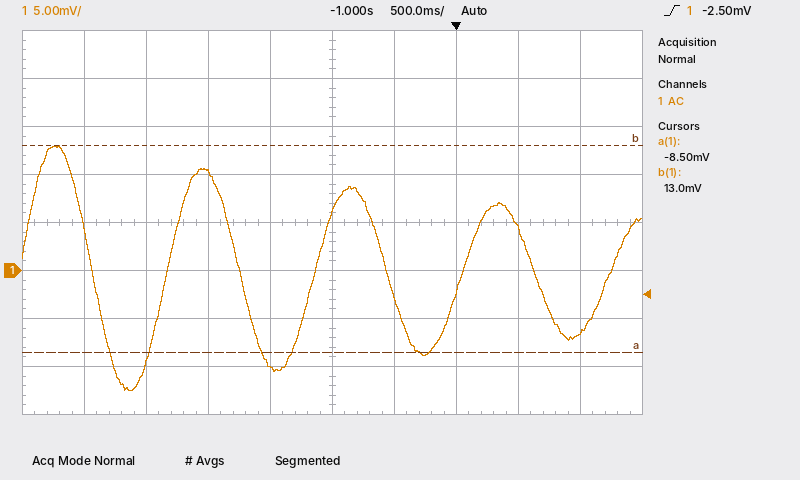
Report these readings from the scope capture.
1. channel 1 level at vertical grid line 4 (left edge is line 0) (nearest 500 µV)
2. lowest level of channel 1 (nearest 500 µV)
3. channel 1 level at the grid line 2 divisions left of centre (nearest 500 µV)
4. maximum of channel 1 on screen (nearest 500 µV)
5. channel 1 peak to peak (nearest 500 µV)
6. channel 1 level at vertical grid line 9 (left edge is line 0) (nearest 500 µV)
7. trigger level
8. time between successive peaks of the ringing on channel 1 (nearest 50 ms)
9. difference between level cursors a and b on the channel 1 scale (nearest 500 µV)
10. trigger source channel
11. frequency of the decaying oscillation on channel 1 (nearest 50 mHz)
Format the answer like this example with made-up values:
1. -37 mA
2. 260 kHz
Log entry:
1. -10.0 mV
2. -12.5 mV
3. 10.0 mV
4. 13.0 mV
5. 25.5 mV
6. -6.5 mV
7. -2.50 mV
8. 1.20 s
9. 21.5 mV
10. channel 1
11. 850 mHz
